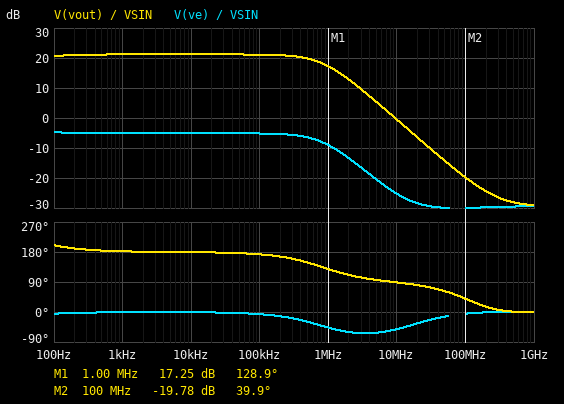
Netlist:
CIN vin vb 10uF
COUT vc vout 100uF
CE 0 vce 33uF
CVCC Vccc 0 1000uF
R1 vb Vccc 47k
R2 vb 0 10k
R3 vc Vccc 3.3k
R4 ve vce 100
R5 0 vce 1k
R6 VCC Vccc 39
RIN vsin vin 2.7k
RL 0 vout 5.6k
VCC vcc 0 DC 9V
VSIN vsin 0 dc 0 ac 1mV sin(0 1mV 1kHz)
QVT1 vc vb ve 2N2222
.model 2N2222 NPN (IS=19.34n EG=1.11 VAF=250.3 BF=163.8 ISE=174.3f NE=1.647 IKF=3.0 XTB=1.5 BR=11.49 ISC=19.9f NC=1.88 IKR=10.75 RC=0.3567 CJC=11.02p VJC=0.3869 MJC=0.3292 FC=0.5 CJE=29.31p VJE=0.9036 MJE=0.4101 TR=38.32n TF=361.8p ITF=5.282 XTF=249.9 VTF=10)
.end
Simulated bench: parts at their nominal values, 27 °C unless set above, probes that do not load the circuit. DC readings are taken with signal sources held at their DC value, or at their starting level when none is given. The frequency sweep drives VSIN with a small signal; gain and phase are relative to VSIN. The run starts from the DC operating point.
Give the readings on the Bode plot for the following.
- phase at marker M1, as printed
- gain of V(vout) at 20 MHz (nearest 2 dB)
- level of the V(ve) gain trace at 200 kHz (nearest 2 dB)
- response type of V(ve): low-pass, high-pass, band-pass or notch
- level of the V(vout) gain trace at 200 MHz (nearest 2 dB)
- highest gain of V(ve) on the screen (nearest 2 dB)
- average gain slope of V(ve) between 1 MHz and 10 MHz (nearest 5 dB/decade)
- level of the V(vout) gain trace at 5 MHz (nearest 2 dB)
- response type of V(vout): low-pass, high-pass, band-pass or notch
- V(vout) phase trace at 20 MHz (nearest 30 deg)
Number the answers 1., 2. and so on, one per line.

1. 128.9 deg
2. -6 dB
3. -6 dB
4. low-pass
5. -24 dB
6. -4 dB
7. -15 dB/decade
8. 6 dB
9. low-pass
10. 90 deg
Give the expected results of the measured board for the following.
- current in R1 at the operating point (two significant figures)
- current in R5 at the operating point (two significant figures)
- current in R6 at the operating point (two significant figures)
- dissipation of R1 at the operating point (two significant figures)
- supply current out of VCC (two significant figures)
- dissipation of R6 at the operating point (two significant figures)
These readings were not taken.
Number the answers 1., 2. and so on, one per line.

1. 160 µA
2. 1.1 mA
3. 1.3 mA
4. 1.2 mW
5. 1.3 mA
6. 63 µW
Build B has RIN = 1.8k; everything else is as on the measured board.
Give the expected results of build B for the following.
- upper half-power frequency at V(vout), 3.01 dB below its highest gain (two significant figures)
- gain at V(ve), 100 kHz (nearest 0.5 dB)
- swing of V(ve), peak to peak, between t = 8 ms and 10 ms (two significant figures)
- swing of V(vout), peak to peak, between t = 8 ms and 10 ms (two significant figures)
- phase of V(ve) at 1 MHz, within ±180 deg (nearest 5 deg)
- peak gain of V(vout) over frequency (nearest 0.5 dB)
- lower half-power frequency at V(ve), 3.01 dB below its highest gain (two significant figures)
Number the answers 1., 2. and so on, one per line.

1. 1.1 MHz
2. -4.0 dB
3. 1.2 mV
4. 26 mV
5. -40 deg
6. 22.0 dB
7. 1.6 Hz
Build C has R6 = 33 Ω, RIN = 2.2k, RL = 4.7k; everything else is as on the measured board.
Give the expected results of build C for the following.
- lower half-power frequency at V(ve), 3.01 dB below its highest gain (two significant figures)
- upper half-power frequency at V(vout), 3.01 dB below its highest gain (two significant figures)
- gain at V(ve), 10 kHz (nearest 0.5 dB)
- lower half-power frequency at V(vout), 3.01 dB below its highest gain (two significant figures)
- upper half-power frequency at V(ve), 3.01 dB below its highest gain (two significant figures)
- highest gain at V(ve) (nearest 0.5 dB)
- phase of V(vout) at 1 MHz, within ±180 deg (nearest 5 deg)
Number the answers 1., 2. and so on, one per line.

1. 1.5 Hz
2. 1.0 MHz
3. -4.5 dB
4. 41 Hz
5. 520 kHz
6. -2.5 dB
7. 135 deg
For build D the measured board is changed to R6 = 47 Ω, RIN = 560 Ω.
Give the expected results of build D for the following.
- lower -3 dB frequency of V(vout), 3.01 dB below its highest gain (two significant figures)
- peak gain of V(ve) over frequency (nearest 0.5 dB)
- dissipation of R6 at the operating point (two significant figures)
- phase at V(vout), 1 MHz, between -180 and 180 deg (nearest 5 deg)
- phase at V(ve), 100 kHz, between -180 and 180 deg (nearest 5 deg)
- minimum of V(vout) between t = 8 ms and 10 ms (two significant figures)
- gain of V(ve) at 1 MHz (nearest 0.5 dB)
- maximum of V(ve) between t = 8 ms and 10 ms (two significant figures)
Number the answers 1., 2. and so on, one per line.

1. 43 Hz
2. -1.0 dB
3. 76 µW
4. 160 deg
5. 0 deg
6. -15 mV
7. -3.0 dB
8. 1.2 V
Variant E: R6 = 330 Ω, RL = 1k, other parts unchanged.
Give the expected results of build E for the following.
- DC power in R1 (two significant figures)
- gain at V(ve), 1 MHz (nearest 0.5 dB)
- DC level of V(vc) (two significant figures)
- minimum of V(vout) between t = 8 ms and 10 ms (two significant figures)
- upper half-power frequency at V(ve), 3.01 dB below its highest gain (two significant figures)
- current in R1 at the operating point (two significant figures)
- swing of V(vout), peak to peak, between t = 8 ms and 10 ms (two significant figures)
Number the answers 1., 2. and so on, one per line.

1. 1.1 mW
2. -6.5 dB
3. 5.1 V
4. -4.2 mV
5. 840 kHz
6. 150 µA
7. 8.4 mV
